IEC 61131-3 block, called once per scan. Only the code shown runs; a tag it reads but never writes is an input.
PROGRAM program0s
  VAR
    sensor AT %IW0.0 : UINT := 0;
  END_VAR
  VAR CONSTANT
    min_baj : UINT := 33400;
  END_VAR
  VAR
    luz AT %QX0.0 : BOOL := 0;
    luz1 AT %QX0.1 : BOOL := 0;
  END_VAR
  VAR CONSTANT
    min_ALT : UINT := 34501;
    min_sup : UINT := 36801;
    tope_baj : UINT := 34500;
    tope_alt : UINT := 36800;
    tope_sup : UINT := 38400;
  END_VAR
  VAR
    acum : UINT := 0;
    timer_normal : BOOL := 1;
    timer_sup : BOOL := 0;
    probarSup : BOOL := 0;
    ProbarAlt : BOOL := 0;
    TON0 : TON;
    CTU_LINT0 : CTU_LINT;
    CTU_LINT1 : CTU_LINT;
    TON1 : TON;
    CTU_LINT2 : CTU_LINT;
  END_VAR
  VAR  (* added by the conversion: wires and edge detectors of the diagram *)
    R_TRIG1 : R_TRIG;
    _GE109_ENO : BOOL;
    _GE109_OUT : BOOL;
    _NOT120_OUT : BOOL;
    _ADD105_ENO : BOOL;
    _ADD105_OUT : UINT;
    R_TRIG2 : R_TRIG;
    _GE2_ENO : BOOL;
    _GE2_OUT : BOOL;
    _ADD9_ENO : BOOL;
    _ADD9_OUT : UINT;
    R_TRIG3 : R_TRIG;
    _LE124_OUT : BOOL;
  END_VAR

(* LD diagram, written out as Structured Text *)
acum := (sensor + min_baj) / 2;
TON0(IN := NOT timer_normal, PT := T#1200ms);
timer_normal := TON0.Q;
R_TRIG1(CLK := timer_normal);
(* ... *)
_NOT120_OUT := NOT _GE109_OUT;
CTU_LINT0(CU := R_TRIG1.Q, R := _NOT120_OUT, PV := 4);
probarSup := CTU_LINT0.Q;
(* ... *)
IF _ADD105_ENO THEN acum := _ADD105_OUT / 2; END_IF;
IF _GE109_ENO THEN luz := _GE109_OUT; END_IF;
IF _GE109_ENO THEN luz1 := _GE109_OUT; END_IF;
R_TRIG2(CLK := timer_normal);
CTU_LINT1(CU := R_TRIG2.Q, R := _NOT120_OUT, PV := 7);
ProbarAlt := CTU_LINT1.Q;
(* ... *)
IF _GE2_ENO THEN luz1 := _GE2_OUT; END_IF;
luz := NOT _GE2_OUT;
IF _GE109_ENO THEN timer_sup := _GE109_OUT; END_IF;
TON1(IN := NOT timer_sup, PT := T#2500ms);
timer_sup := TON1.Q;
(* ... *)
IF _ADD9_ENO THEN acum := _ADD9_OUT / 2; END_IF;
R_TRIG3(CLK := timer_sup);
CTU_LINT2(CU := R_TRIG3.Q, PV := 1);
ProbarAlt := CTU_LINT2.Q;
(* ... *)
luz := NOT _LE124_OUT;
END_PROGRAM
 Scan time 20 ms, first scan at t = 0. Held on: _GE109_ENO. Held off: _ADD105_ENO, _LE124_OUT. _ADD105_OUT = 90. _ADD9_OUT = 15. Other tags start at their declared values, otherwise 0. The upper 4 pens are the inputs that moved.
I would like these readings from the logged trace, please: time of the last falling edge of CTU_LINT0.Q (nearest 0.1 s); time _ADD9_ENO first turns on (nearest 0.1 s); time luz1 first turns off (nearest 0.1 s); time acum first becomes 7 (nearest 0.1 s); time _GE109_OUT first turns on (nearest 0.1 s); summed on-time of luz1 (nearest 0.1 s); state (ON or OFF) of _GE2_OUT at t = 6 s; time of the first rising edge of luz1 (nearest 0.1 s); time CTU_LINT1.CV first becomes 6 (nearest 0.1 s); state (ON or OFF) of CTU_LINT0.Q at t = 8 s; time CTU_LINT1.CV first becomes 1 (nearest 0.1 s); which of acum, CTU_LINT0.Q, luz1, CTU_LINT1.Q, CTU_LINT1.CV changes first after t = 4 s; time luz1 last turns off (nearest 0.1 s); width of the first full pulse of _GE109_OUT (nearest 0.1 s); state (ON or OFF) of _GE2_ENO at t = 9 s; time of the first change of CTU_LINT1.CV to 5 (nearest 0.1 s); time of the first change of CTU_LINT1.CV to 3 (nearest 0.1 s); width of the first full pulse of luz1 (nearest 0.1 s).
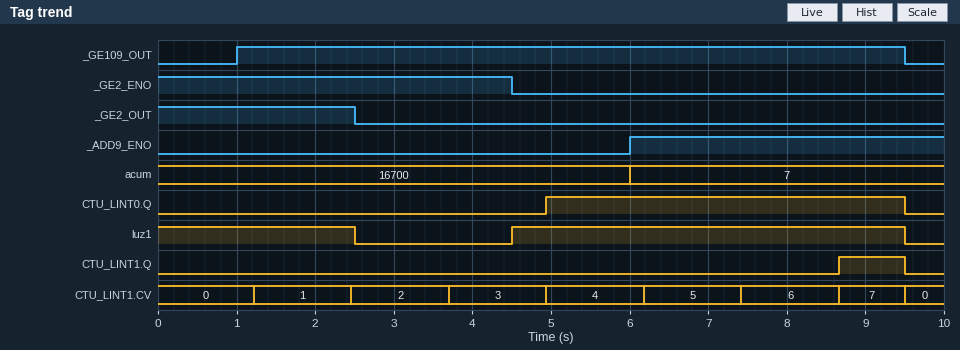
9.5 s
6.0 s
2.5 s
6.0 s
1.0 s
7.5 s
OFF
4.5 s
7.4 s
ON
1.2 s
luz1
9.5 s
8.5 s
OFF
6.2 s
3.7 s
5.0 s
